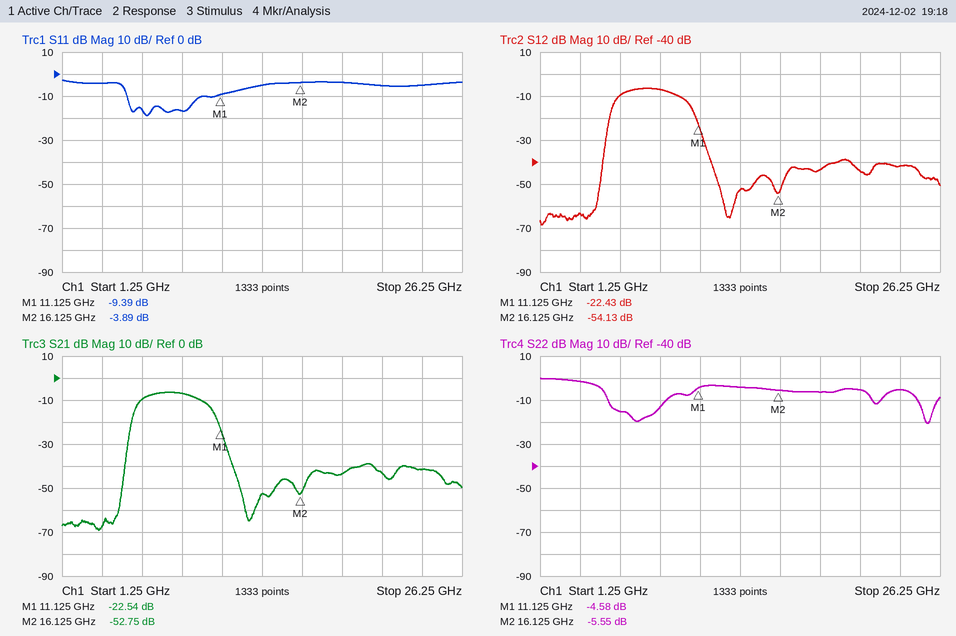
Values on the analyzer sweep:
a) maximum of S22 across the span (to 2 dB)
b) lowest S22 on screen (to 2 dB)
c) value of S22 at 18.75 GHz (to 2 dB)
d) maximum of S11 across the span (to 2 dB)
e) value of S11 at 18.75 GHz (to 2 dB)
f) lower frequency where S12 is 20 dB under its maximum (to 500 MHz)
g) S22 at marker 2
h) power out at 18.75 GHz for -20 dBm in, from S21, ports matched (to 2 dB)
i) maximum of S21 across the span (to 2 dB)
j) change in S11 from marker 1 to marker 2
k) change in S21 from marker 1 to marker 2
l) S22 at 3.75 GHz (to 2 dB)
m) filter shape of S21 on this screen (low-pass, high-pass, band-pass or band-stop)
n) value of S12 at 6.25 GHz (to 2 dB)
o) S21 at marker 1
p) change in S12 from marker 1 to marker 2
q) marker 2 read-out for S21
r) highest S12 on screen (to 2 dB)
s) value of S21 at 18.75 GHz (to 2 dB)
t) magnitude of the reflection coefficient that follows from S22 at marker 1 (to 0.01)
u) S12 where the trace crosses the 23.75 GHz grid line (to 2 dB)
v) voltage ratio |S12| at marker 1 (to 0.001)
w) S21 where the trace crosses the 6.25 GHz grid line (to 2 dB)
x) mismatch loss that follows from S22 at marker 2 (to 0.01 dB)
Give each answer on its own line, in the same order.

0 dB
-20 dB
-6 dB
-2 dB
-4 dB
5.5 GHz
-5.55 dB
-64 dBm
-6 dB
5.50 dB
-30.21 dB
-2 dB
band-pass
-10 dB
-22.54 dB
-31.70 dB
-52.75 dB
-6 dB
-44 dB
0.59
-42 dB
0.076
-10 dB
1.42 dB
